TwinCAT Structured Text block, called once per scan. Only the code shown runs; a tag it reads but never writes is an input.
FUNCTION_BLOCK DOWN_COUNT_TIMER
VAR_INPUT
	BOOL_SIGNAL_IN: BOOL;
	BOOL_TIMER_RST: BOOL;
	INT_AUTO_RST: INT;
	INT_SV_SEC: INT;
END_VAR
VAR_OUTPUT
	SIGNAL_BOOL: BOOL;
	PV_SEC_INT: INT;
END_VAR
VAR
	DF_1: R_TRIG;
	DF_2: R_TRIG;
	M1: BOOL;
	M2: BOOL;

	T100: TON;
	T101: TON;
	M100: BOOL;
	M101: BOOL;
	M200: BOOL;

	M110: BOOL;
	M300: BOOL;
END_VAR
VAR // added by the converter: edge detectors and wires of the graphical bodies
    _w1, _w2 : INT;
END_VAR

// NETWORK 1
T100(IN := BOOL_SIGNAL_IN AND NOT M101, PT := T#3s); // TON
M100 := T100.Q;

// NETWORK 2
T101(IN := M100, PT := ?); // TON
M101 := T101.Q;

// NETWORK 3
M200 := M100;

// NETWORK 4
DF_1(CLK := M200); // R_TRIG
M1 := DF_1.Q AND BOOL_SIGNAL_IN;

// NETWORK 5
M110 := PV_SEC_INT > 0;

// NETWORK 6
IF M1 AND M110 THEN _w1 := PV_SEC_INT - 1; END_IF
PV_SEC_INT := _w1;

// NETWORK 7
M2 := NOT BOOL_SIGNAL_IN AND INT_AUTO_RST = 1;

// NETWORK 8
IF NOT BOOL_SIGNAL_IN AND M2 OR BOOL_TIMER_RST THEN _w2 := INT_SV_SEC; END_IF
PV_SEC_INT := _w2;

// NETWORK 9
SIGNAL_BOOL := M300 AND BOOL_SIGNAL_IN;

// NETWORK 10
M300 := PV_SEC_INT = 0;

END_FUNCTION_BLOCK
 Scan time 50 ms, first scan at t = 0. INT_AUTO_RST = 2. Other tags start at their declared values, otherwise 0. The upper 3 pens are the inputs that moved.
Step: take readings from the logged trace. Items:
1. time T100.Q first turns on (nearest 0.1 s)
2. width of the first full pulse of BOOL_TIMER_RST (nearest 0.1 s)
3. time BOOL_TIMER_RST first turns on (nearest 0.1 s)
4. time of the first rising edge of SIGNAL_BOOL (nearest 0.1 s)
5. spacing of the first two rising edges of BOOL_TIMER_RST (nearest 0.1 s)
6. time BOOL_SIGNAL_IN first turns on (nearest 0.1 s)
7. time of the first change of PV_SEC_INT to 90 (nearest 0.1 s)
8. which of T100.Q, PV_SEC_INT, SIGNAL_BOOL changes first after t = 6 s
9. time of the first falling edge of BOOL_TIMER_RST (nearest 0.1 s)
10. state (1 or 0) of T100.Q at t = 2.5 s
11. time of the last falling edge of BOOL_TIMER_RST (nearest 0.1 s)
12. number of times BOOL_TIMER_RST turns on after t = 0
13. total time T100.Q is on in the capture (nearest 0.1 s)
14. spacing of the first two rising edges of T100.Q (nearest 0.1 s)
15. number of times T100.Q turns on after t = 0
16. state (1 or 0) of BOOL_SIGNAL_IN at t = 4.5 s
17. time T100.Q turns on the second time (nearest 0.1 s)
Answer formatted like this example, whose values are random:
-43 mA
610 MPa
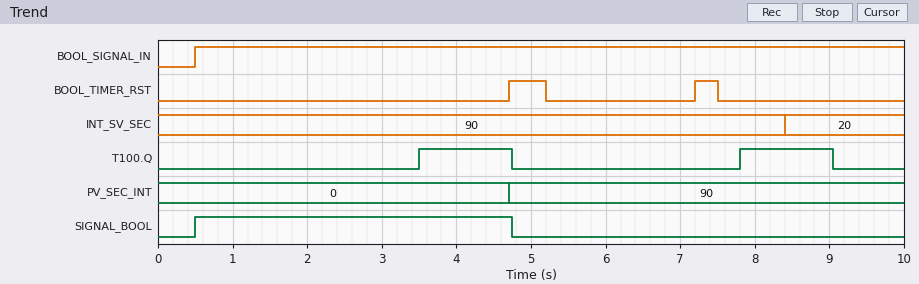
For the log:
3.5 s
0.5 s
4.7 s
0.5 s
2.5 s
0.5 s
4.7 s
T100.Q
5.2 s
0
7.5 s
2
2.5 s
4.3 s
2
1
7.8 s
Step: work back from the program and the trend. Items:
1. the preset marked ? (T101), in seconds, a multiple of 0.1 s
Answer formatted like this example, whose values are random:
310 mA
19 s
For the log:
1.2 s
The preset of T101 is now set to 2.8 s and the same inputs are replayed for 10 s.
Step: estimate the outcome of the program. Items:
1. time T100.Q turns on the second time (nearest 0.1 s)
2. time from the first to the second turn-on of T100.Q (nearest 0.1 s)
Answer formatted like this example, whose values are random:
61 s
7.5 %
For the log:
9.4 s
5.9 s
